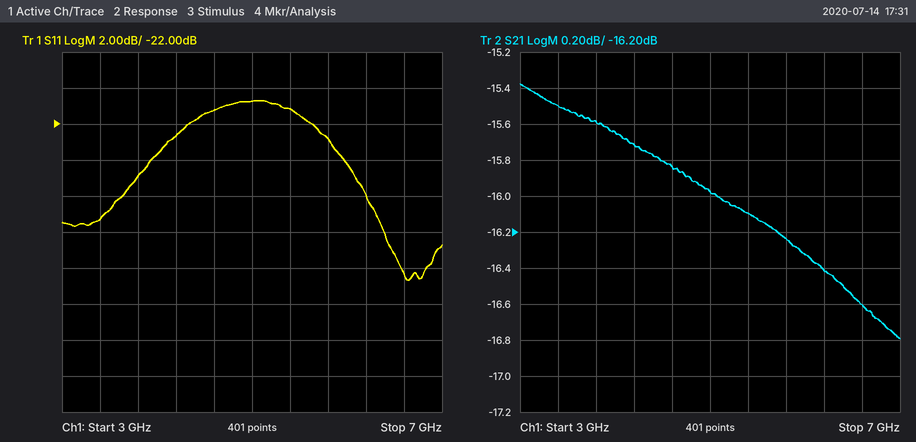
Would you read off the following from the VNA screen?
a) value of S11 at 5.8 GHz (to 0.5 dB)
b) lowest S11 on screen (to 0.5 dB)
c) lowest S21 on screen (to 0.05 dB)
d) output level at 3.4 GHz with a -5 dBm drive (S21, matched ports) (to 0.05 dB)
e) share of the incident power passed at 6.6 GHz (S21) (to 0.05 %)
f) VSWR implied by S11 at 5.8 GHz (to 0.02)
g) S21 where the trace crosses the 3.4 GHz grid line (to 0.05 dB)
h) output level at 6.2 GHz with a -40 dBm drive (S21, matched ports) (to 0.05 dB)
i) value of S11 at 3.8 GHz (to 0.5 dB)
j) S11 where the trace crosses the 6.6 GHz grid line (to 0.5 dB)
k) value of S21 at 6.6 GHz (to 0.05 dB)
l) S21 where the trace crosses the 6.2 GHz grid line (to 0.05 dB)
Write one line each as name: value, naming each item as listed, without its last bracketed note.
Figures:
value of S11 at 5.8 GHz: -23.0 dB
lowest S11 on screen: -30.5 dB
lowest S21 on screen: -16.80 dB
output level at 3.4 GHz with a -5 dBm drive (S21, matched ports): -20.50 dBm
share of the incident power passed at 6.6 GHz (S21): 2.20 %
VSWR implied by S11 at 5.8 GHz: 1.16
S21 where the trace crosses the 3.4 GHz grid line: -15.50 dB
output level at 6.2 GHz with a -40 dBm drive (S21, matched ports): -56.40 dBm
value of S11 at 3.8 GHz: -25.0 dB
S11 where the trace crosses the 6.6 GHz grid line: -30.5 dB
value of S21 at 6.6 GHz: -16.60 dB
S21 where the trace crosses the 6.2 GHz grid line: -16.40 dB
